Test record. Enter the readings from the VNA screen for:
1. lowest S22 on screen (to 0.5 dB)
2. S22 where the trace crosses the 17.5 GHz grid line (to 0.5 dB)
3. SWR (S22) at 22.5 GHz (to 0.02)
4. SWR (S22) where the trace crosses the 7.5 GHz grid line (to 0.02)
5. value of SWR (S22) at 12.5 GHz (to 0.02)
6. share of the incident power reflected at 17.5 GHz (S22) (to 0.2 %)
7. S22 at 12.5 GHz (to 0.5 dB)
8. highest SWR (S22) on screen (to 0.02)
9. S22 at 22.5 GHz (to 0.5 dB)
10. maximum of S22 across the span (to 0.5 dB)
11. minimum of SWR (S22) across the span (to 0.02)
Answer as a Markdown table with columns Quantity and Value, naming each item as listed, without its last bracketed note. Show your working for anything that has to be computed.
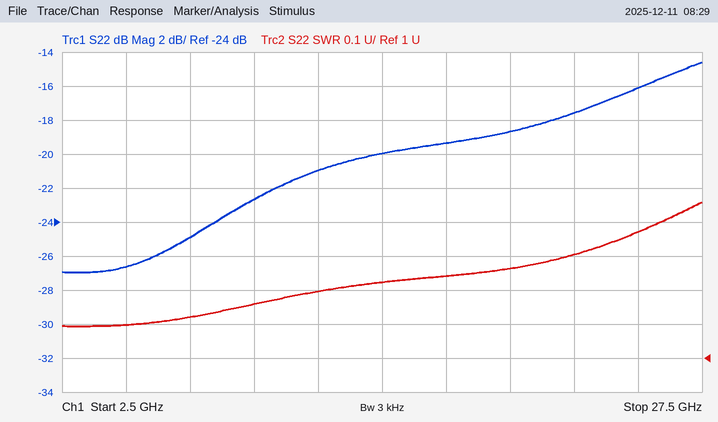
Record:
| Quantity | Value |
|---|---|
| lowest S22 on screen | -27.0 dB |
| S22 where the trace crosses the 17.5 GHz grid line | -19.5 dB |
| SWR (S22) at 22.5 GHz | 1.30 |
| SWR (S22) where the trace crosses the 7.5 GHz grid line | 1.12 |
| value of SWR (S22) at 12.5 GHz | 1.20 |
| share of the incident power reflected at 17.5 GHz (S22) | 10^(-19.5/10) ≈ 1.12 %, so 1.2 % to the nearest 0.2 % |
| S22 at 12.5 GHz | -21.0 dB |
| highest SWR (S22) on screen | 1.46 |
| S22 at 22.5 GHz | -17.5 dB |
| maximum of S22 across the span | -14.5 dB |
| minimum of SWR (S22) across the span | 1.10 |
